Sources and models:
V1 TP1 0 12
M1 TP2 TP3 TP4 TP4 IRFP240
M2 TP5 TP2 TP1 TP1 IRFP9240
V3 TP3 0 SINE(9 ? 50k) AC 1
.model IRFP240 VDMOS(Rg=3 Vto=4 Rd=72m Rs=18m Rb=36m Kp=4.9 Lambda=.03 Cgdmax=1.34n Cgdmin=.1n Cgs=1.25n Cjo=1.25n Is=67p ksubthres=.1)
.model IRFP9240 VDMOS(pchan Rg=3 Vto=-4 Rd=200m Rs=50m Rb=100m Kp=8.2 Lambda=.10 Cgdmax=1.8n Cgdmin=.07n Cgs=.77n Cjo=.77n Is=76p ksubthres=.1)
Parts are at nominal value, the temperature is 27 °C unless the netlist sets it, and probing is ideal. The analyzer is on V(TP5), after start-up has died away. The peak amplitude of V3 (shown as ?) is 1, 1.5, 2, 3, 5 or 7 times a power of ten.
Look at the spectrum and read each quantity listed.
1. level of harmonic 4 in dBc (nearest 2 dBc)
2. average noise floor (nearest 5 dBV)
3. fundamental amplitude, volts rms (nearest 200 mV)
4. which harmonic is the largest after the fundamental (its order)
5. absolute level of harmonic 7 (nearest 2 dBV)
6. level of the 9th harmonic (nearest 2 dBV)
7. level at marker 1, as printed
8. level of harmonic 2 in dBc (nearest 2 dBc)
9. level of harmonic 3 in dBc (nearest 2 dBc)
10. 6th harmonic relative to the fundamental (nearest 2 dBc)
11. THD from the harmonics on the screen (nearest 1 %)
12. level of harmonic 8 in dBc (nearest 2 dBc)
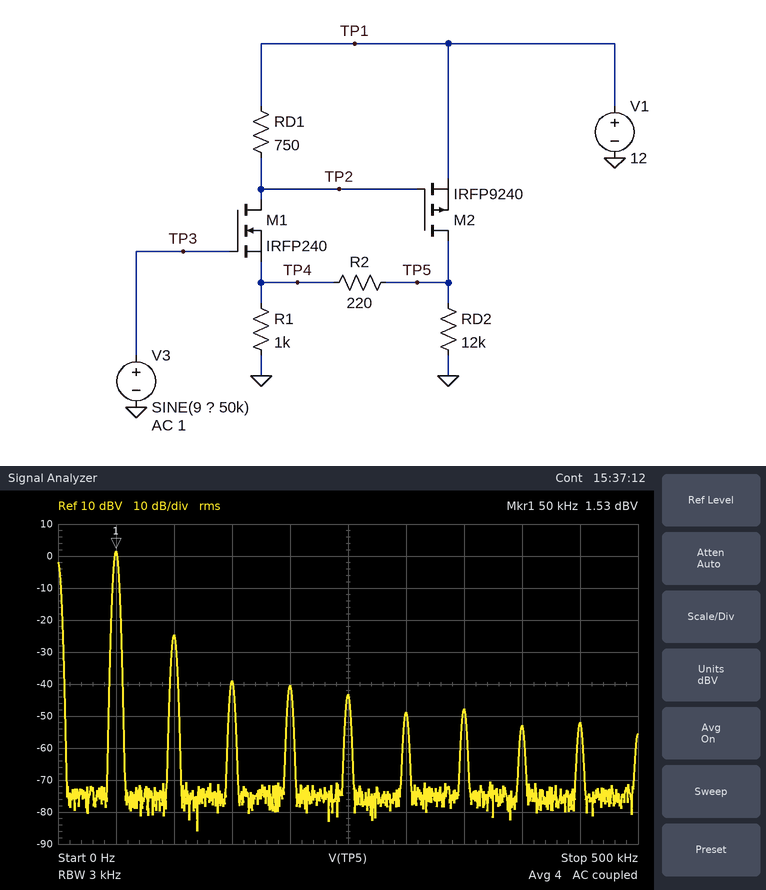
-42 dBc
-75 dBV
1.2 V
2
-48 dBV
-52 dBV
1.53 dBV
-26 dBc
-40 dBc
-50 dBc
5 %
-54 dBc
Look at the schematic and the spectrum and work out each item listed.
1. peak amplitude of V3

1.5 V
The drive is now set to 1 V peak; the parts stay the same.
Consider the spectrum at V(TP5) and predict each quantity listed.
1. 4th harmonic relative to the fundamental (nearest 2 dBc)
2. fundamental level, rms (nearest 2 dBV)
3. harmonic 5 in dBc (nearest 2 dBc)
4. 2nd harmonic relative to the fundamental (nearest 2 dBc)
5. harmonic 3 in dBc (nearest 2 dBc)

-50 dBc
-2 dBV
-48 dBc
-28 dBc
-38 dBc
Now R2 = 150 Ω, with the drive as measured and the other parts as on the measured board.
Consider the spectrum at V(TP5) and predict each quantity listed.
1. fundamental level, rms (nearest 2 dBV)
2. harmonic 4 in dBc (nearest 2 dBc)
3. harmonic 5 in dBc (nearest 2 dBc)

2 dBV
-44 dBc
-48 dBc
